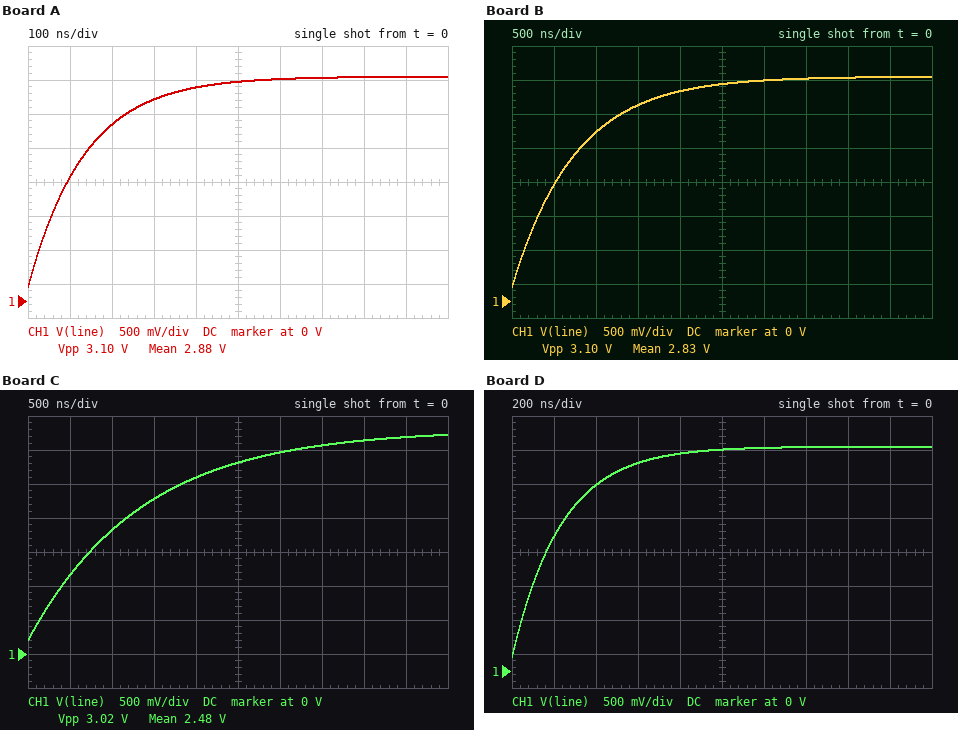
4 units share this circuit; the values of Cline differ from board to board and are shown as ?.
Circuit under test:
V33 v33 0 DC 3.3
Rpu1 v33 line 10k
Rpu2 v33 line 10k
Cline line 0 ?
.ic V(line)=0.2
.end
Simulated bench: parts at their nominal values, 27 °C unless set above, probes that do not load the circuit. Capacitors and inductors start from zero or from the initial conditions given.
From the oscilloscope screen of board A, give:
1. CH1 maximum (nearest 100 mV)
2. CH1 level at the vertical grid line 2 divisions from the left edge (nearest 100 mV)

3.3 V
2.6 V
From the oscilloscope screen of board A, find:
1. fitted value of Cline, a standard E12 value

27 pF
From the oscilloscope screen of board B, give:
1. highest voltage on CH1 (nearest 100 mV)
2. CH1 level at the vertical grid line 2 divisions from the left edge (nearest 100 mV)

3.3 V
2.5 V
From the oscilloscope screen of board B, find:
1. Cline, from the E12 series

150 pF
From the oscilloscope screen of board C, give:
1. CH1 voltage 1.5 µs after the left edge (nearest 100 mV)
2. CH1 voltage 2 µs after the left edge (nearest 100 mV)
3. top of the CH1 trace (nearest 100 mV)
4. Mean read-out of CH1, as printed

2.3 V
2.6 V
3.2 V
2.48 V
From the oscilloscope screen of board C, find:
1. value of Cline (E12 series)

270 pF
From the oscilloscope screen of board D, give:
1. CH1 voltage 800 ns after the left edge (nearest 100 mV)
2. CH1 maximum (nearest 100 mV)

3.2 V
3.3 V
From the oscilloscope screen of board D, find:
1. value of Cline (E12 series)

47 pF
